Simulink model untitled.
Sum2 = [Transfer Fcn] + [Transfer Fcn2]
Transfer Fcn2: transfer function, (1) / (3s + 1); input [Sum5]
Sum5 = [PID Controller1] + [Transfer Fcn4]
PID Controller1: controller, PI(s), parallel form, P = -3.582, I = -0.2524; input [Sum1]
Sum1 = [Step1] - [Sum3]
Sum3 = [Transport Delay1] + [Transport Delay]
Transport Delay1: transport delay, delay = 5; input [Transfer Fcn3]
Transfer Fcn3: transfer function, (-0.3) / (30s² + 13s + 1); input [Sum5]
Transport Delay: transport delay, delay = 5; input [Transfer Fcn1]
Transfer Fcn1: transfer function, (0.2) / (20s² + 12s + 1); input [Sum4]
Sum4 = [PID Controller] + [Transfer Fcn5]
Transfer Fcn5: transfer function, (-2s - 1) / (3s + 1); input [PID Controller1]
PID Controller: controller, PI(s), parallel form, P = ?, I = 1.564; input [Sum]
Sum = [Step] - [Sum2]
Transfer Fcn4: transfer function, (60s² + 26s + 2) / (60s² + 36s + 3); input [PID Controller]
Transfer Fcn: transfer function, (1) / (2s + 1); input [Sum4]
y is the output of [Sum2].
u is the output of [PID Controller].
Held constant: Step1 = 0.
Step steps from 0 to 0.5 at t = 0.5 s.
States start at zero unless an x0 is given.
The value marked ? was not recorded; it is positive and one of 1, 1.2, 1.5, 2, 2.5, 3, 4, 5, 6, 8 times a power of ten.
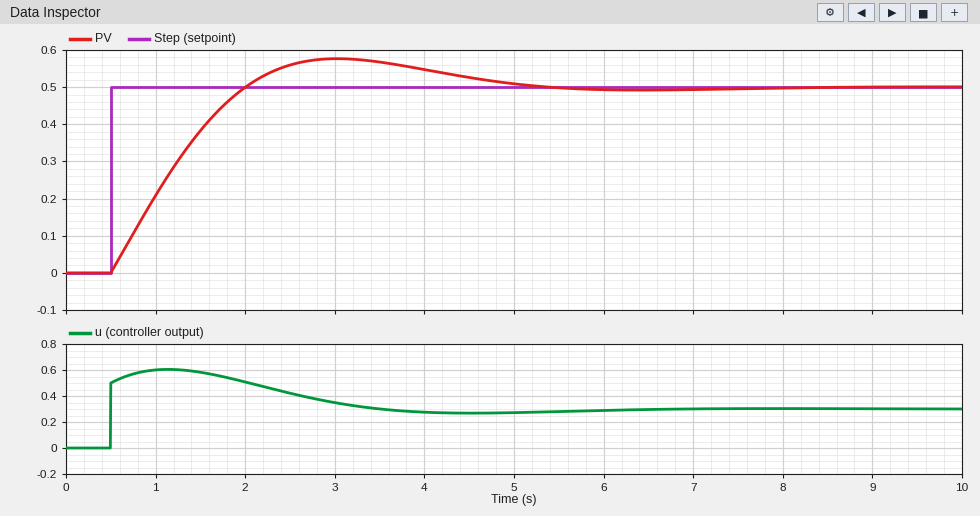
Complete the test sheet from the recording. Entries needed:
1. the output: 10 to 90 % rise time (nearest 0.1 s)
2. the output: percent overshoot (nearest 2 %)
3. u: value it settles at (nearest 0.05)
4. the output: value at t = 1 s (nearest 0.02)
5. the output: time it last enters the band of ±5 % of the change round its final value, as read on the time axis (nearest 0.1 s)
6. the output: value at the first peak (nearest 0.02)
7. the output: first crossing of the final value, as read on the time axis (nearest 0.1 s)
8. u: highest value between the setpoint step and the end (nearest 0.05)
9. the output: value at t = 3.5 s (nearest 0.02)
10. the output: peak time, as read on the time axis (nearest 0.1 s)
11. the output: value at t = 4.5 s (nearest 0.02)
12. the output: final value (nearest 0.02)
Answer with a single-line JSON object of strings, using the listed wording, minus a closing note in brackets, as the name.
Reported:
{"the output: 10 to 90 % rise time": "1.1 s", "the output: percent overshoot": "16 %", "u: value it settles at": "0.30", "the output: value at t = 1 s": "0.20", "the output: time it last enters the band of ±5 % of the change round its final value, as read on the time axis": "4.5 s", "the output: value at the first peak": "0.58", "the output: first crossing of the final value, as read on the time axis": "2.0 s", "u: highest value between the setpoint step and the end": "0.60", "the output: value at t = 3.5 s": "0.56", "the output: peak time, as read on the time axis": "3.0 s", "the output: value at t = 4.5 s": "0.52", "the output: final value": "0.50"}
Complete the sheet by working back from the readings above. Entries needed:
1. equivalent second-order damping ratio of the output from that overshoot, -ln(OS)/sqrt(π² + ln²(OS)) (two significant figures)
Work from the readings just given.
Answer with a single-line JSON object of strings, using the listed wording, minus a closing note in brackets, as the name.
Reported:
{"equivalent second-order damping ratio of the output from that overshoot, -ln(OS)/sqrt(π² + ln²(OS))": "0.50"}
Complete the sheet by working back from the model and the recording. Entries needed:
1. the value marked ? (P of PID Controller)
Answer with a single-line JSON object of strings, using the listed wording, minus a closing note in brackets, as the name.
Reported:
{"the value marked ?": "1"}
